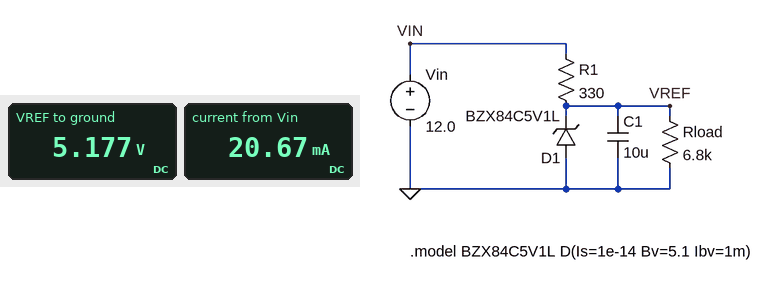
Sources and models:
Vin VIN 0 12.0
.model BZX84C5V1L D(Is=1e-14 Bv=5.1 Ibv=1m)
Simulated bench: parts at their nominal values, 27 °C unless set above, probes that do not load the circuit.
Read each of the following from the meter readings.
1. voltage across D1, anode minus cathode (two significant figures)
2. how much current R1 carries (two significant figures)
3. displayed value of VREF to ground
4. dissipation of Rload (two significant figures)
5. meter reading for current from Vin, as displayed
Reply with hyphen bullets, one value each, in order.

- -5.2 V
- 21 mA
- 5.177 V
- 3.9 mW
- 20.67 mA
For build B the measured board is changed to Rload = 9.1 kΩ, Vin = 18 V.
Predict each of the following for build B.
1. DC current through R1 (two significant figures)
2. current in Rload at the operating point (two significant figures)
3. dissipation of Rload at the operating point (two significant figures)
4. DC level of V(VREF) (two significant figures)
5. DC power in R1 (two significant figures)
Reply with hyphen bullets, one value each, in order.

- 39 mA
- 570 µA
- 3.0 mW
- 5.2 V
- 500 mW
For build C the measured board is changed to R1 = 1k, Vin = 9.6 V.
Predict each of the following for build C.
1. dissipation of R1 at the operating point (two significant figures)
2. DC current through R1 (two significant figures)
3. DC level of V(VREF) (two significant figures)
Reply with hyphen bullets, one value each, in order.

- 20 mW
- 4.5 mA
- 5.1 V
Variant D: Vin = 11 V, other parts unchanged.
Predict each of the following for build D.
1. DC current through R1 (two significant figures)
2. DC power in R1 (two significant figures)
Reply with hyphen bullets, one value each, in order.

- 18 mA
- 100 mW
